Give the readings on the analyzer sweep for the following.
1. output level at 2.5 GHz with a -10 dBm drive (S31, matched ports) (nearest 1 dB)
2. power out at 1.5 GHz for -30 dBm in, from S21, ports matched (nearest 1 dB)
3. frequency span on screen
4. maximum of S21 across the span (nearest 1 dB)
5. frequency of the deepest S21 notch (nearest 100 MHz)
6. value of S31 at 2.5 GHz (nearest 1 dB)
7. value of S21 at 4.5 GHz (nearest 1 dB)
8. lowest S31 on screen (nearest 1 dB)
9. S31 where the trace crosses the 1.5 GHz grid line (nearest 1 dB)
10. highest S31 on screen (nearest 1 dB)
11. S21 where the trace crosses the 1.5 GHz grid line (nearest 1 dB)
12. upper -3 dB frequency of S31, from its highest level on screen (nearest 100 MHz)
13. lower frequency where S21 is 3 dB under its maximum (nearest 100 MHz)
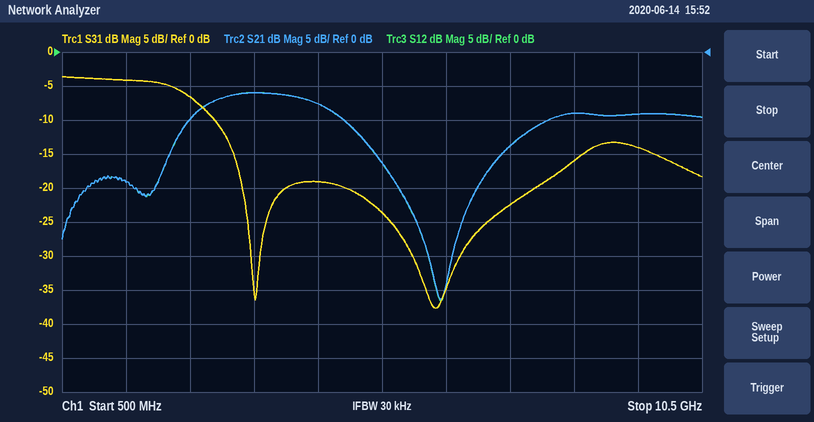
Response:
-17 dBm
-49 dBm
10 GHz
-6 dB
6.4 GHz
-7 dB
-8 dB
-38 dB
-4 dB
-4 dB
-19 dB
2.5 GHz
2.6 GHz
